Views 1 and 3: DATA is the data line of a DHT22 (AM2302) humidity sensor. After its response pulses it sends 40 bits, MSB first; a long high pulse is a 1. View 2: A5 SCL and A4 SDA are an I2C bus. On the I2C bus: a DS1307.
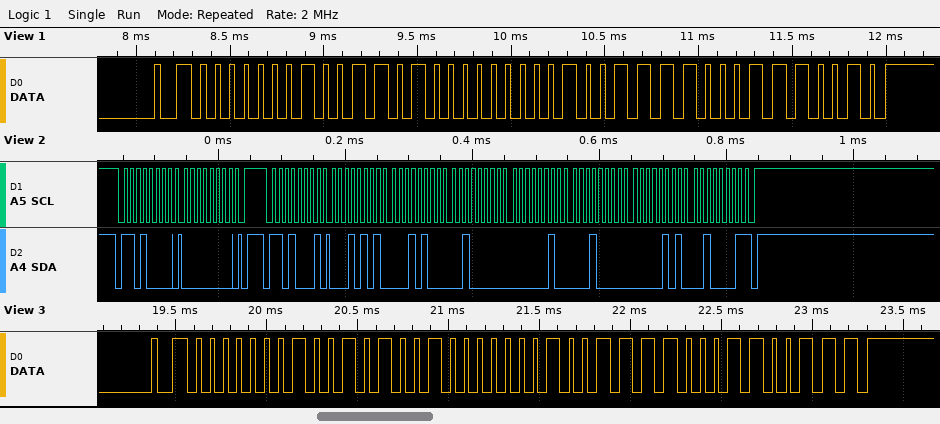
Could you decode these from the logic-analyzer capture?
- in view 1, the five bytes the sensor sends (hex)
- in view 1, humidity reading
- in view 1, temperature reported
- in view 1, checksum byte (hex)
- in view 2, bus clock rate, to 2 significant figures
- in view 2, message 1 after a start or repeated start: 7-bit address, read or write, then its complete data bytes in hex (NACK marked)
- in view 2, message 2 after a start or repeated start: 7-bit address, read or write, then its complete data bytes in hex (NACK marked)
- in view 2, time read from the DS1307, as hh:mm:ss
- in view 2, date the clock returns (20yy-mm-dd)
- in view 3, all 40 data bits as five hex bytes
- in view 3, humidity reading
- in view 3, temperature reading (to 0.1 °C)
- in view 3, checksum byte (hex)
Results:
01 34 01 3C 72
30.8 %
31.6 °C
0x72
100 kHz
0x68 write: 00
0x68 read: 15 14 20 02 10 05 21 NACK
20:14:15
2021-05-10
01 29 01 3C 67
29.7 %
31.6 °C
0x67
